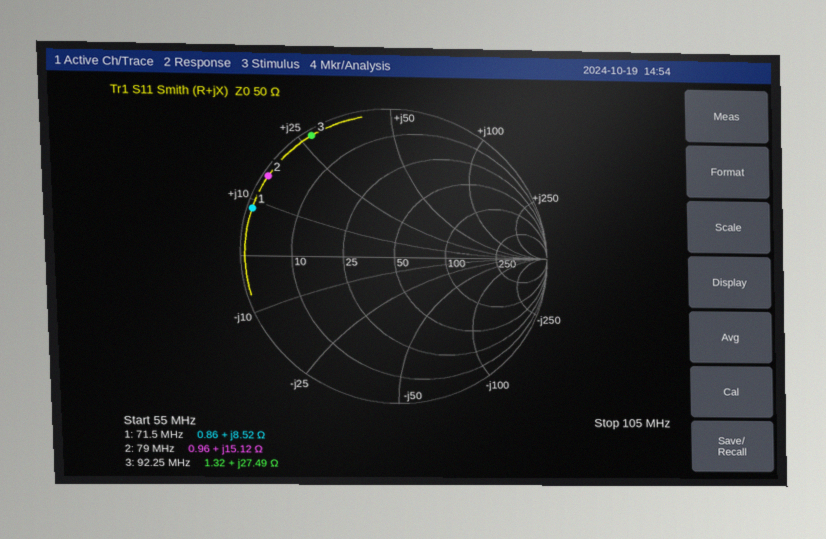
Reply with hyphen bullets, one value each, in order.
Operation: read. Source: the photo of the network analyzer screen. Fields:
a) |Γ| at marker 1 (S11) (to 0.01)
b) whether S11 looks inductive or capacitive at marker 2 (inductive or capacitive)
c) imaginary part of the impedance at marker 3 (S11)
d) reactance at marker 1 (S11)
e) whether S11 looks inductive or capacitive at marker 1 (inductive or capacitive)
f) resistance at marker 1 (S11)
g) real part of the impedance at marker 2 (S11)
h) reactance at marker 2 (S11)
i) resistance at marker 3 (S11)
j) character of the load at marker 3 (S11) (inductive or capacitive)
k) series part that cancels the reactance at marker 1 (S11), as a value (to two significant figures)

- 0.97
- inductive
- +27.49 Ω
- +8.52 Ω
- inductive
- 0.86 Ω
- 0.96 Ω
- +15.12 Ω
- 1.32 Ω
- inductive
- 260 pF
